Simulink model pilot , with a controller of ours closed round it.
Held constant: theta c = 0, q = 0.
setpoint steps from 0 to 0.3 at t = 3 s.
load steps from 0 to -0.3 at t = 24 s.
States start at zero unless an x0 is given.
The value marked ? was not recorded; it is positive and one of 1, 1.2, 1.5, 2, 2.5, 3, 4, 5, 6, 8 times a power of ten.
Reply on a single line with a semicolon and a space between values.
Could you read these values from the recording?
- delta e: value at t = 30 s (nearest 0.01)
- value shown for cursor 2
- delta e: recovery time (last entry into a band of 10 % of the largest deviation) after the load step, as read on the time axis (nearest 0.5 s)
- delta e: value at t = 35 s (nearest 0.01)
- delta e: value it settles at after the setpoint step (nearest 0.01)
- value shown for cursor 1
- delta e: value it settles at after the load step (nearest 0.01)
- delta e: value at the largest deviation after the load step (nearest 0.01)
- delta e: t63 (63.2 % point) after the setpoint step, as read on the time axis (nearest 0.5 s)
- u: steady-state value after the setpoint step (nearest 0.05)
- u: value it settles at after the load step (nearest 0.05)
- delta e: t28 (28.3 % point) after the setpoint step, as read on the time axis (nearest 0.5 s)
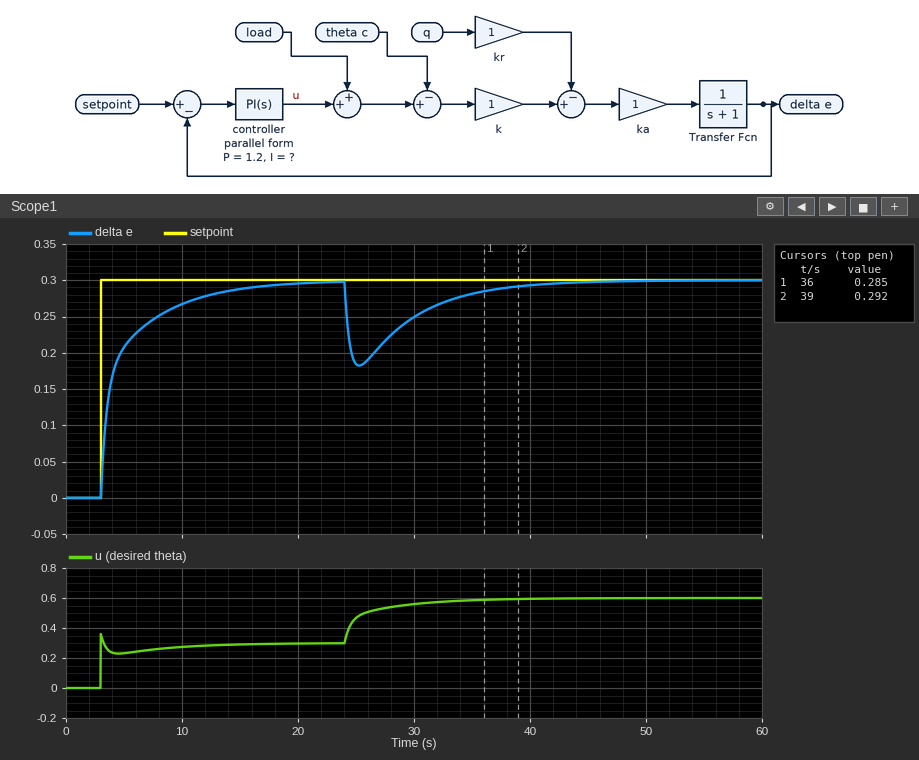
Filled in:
0.25; 0.292; 37.5 s; 0.28; 0.30; 0.285; 0.30; 0.18; 4.5 s; 0.30; 0.60; 3.5 s
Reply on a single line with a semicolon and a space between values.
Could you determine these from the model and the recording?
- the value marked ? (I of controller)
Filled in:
0.4
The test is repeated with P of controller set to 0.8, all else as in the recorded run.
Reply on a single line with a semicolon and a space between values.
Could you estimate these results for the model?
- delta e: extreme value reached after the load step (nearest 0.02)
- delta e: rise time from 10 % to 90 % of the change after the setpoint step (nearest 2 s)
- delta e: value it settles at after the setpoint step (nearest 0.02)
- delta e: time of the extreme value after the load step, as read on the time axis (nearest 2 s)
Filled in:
0.16; 6 s; 0.30; 26 s
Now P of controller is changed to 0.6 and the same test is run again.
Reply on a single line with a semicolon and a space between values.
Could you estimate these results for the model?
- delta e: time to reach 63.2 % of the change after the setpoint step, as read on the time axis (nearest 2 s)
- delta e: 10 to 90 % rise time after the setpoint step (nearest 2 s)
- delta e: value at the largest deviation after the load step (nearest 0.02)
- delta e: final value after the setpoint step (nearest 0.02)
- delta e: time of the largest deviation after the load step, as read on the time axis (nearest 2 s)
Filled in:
6 s; 6 s; 0.16; 0.30; 26 s
